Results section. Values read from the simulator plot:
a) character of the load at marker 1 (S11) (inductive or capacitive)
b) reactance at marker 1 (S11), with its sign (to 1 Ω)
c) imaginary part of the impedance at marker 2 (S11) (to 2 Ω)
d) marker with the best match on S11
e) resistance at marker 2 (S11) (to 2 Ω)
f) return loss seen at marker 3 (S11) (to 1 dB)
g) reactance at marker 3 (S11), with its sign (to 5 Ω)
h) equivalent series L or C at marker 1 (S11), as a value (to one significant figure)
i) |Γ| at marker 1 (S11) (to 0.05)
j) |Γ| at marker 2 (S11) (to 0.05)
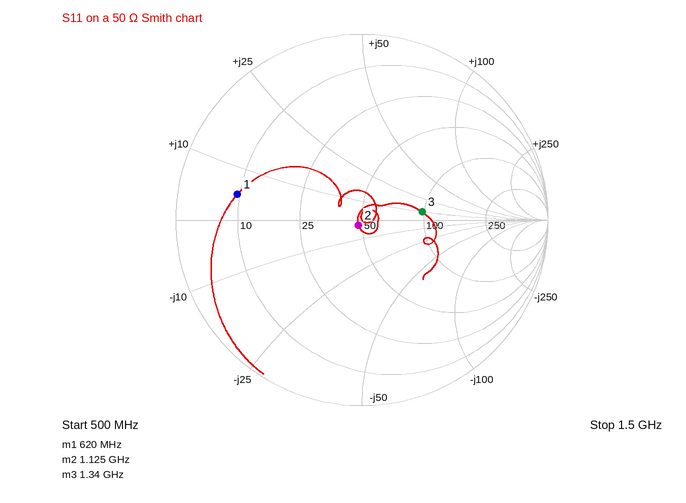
inductive
+5 Ω
-2 Ω
marker 2
48 Ω
10 dB
+10 Ω
1 nH
0.70
0.05
